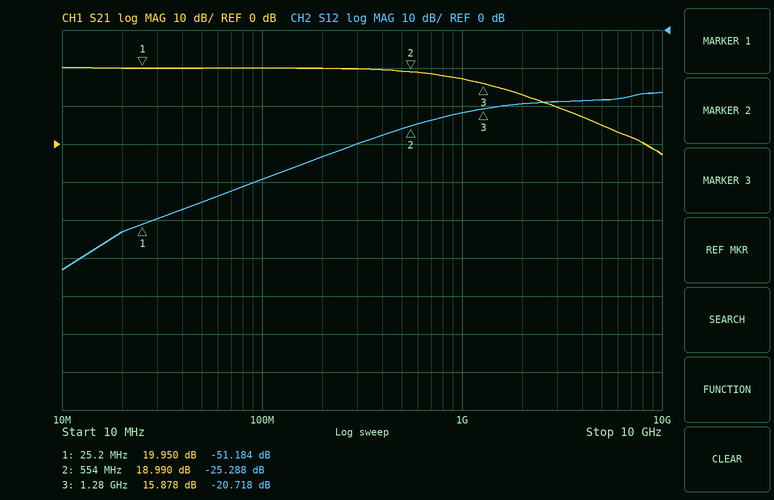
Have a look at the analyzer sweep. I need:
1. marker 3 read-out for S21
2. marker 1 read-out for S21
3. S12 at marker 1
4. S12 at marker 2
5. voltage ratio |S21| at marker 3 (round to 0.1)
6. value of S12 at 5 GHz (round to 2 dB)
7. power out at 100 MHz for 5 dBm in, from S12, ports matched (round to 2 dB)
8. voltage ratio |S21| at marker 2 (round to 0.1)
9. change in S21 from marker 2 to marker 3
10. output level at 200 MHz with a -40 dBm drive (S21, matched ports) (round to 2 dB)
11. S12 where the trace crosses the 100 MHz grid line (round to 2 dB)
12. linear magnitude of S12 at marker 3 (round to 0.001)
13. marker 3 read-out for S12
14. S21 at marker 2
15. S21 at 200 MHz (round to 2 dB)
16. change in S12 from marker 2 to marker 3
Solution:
15.878 dB
19.950 dB
-51.184 dB
-25.288 dB
6.2
-18 dB
-34 dBm
8.9
-3.112 dB
-20 dBm
-40 dB
0.092
-20.718 dB
18.990 dB
20 dB
4.570 dB
